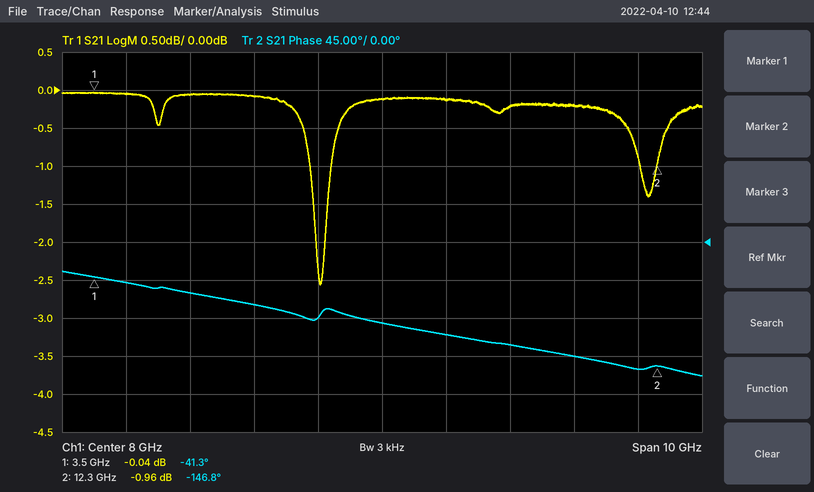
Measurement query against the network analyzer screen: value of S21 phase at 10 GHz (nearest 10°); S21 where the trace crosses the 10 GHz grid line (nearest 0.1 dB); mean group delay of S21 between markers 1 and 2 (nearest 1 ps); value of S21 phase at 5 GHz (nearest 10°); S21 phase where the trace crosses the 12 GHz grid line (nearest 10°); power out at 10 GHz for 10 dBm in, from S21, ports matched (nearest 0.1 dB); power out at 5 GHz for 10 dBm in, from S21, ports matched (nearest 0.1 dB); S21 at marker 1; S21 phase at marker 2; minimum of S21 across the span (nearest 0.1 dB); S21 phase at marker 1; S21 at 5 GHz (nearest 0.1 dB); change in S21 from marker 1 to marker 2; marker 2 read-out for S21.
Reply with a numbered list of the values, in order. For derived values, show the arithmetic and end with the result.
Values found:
1. -120°
2. -0.2 dB
3. −(-146.8° − (-41.3°))/(360° × 8.8 GHz) ≈ 33 ps
4. -60°
5. -150°
6. 10 dBm + (-0.2 dB) = 9.8 dBm
7. 10 dBm + (-0.1 dB) = 9.9 dBm
8. -0.04 dB
9. -146.8°
10. -2.6 dB
11. -41.3°
12. -0.1 dB
13. -0.96 − (-0.04) = -0.92 dB
14. -0.96 dB
